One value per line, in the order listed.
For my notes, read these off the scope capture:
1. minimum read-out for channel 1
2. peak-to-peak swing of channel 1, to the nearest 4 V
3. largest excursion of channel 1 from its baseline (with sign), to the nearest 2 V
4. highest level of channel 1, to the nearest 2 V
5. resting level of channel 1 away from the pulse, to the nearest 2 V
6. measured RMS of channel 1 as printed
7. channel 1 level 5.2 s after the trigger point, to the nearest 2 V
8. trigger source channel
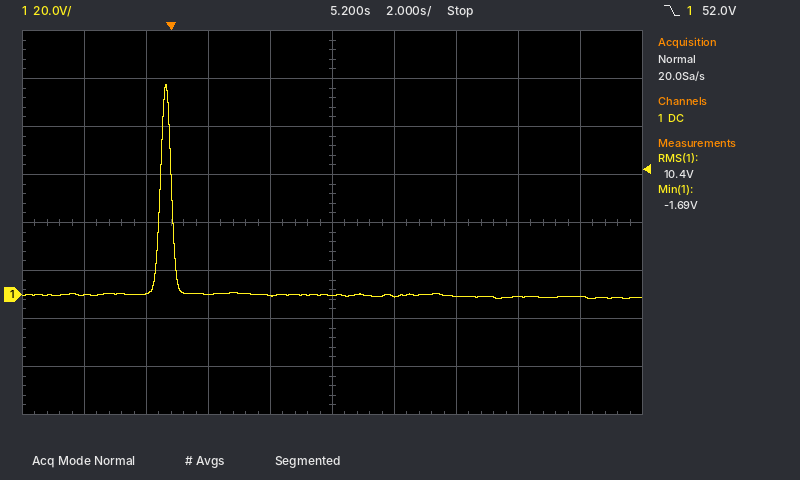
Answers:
-1.69 V
88 V
+88 V
88 V
0 V
10.4 V
0 V
channel 1
